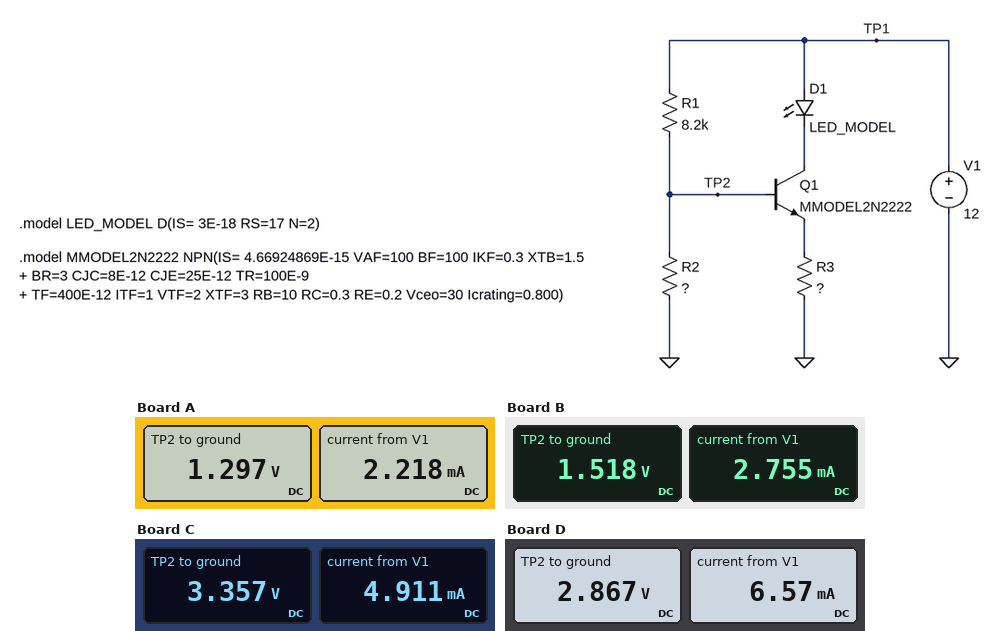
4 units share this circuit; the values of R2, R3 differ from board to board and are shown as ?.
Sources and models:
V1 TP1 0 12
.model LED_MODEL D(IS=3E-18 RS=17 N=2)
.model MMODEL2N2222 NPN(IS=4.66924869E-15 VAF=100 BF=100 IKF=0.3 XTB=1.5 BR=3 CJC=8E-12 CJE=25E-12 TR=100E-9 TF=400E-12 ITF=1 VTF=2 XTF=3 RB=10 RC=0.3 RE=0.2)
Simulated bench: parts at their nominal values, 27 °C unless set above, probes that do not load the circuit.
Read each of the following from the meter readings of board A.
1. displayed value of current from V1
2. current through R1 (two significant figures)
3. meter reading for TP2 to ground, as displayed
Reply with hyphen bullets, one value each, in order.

- 2.218 mA
- 1.3 mA
- 1.297 V
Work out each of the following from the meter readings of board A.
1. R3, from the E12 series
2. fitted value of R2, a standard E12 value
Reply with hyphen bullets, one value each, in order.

- 680 Ω
- 1 kΩ
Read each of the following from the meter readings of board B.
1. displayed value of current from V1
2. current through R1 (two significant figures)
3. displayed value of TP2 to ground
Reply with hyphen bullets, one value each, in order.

- 2.755 mA
- 1.3 mA
- 1.518 V
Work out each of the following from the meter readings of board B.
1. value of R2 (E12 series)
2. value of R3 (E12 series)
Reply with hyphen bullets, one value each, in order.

- 1.2 kΩ
- 560 Ω
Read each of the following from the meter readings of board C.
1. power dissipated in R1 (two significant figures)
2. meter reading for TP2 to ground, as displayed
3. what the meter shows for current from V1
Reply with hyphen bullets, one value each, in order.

- 9.1 mW
- 3.357 V
- 4.911 mA
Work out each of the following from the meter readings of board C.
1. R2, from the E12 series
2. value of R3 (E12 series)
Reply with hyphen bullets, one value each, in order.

- 3.3 kΩ
- 680 Ω
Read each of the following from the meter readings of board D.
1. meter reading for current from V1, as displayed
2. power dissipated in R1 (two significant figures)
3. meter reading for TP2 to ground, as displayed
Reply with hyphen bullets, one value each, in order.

- 6.57 mA
- 10 mW
- 2.867 V
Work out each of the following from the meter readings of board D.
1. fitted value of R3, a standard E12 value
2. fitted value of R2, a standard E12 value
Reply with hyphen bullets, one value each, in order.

- 390 Ω
- 2.7 kΩ
